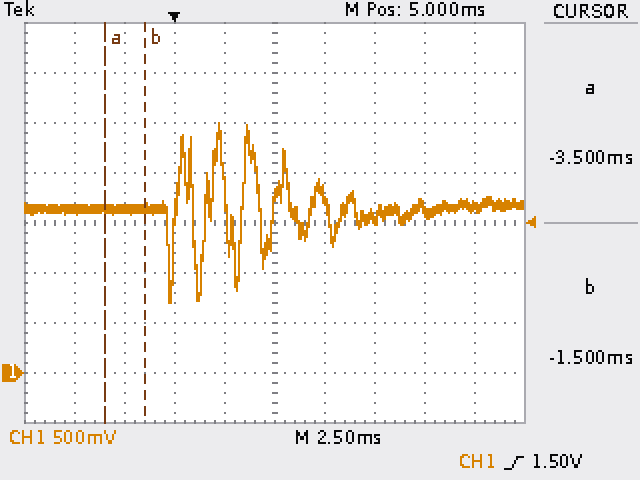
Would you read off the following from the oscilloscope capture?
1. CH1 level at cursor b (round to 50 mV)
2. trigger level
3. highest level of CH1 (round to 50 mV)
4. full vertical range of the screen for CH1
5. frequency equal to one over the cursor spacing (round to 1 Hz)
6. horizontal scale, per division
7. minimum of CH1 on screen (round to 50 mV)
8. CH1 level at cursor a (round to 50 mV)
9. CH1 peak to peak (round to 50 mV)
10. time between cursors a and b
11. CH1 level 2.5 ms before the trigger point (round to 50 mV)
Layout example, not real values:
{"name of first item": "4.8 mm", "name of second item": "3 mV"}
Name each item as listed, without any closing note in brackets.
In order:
{"CH1 level at cursor b": "1.65 V", "trigger level": "1.50 V", "highest level of CH1": "2.50 V", "full vertical range of the screen for CH1": "4 V", "frequency equal to one over the cursor spacing": "500 Hz", "horizontal scale, per division": "2.5 ms", "minimum of CH1 on screen": "700 mV", "CH1 level at cursor a": "1.65 V", "CH1 peak to peak": "1.80 V", "time between cursors a and b": "2.00 ms", "CH1 level 2.5 ms before the trigger point": "1.65 V"}
